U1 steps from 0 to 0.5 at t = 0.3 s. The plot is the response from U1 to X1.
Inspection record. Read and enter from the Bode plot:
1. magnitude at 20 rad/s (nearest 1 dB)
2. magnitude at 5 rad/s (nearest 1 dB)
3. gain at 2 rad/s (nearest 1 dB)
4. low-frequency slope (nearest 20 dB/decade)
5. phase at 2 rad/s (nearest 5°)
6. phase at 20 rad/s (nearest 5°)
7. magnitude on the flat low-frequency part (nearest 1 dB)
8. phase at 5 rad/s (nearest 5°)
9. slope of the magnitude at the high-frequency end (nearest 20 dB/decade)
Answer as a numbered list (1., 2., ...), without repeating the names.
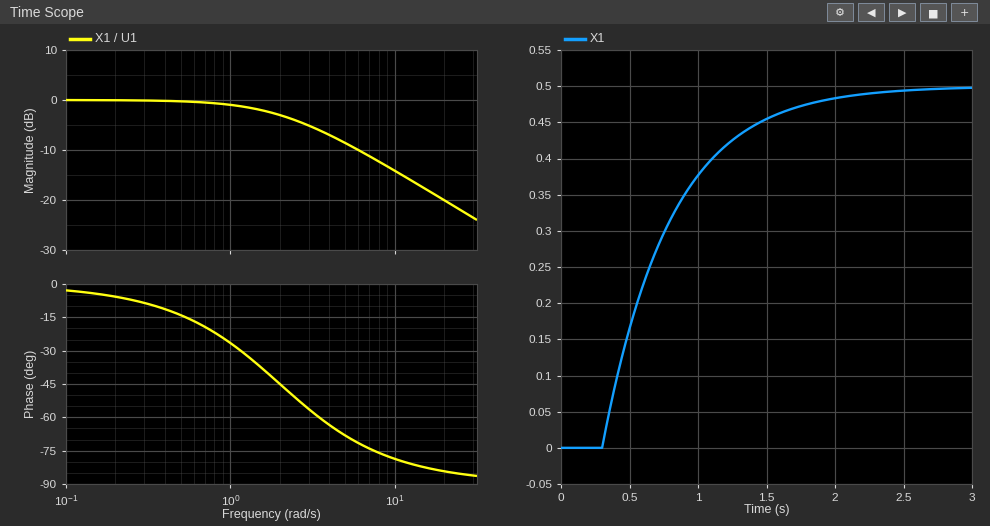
1. -20 dB
2. -9 dB
3. -3 dB
4. 0 dB/decade
5. -45°
6. -85°
7. 0 dB
8. -70°
9. -20 dB/decade
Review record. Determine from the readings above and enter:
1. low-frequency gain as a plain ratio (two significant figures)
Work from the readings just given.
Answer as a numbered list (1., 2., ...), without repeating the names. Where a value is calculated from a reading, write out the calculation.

1. 10^(0 / 20) = 1.0
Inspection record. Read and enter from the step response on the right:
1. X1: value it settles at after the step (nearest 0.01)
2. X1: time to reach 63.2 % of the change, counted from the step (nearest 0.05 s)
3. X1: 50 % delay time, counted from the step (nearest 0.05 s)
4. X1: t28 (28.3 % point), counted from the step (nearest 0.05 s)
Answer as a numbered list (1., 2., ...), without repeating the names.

1. 0.50
2. 0.50 s
3. 0.35 s
4. 0.15 s
